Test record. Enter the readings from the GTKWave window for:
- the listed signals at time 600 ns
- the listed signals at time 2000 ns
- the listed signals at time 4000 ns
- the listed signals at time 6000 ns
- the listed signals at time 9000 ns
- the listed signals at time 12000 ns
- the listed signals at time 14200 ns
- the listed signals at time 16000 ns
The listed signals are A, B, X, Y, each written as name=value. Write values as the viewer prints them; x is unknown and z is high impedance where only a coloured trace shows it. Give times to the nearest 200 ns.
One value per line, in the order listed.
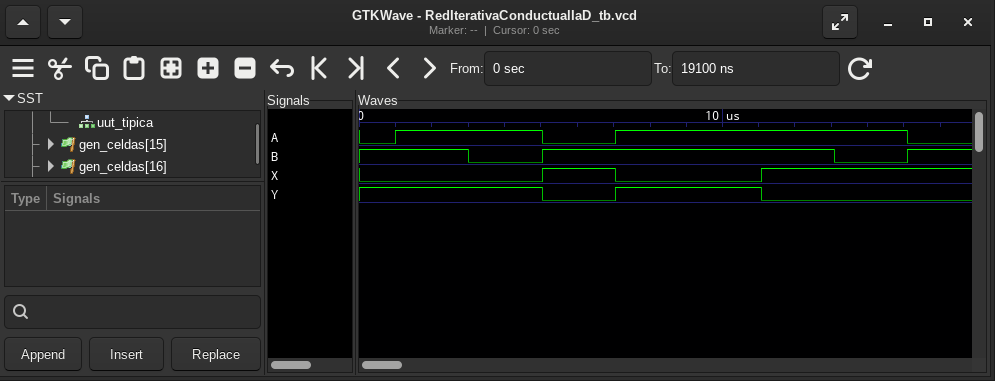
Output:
A=0, B=1, X=0, Y=1
A=1, B=1, X=0, Y=1
A=1, B=0, X=0, Y=1
A=0, B=1, X=1, Y=0
A=1, B=1, X=0, Y=1
A=1, B=1, X=1, Y=0
A=1, B=0, X=1, Y=0
A=0, B=1, X=1, Y=0
